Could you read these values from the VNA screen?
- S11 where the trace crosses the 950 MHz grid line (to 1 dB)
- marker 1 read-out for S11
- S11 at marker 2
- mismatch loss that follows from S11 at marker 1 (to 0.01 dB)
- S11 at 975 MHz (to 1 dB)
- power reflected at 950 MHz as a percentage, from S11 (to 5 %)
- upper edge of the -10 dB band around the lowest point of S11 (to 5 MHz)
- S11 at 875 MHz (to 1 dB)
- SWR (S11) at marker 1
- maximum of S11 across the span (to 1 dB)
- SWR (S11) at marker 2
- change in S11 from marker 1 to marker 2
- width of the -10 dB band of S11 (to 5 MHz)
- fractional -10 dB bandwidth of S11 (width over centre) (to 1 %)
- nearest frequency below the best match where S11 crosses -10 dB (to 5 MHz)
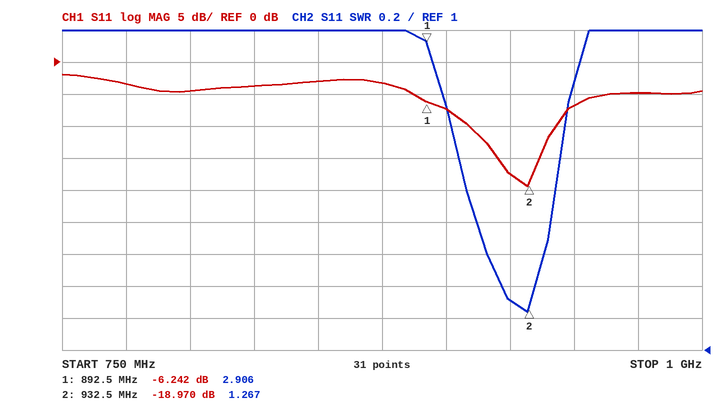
-7 dB
-6.242 dB
-18.970 dB
1.18 dB
-5 dB
20 %
945 MHz
-3 dB
2.906
-2 dB
1.267
-12.728 dB
35 MHz
4 %
910 MHz
